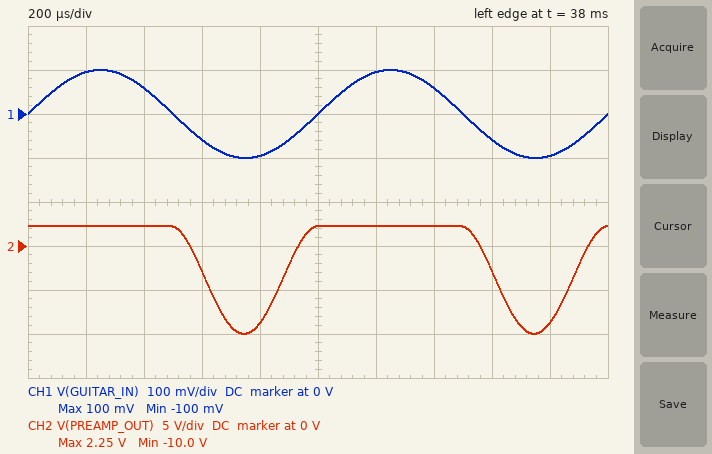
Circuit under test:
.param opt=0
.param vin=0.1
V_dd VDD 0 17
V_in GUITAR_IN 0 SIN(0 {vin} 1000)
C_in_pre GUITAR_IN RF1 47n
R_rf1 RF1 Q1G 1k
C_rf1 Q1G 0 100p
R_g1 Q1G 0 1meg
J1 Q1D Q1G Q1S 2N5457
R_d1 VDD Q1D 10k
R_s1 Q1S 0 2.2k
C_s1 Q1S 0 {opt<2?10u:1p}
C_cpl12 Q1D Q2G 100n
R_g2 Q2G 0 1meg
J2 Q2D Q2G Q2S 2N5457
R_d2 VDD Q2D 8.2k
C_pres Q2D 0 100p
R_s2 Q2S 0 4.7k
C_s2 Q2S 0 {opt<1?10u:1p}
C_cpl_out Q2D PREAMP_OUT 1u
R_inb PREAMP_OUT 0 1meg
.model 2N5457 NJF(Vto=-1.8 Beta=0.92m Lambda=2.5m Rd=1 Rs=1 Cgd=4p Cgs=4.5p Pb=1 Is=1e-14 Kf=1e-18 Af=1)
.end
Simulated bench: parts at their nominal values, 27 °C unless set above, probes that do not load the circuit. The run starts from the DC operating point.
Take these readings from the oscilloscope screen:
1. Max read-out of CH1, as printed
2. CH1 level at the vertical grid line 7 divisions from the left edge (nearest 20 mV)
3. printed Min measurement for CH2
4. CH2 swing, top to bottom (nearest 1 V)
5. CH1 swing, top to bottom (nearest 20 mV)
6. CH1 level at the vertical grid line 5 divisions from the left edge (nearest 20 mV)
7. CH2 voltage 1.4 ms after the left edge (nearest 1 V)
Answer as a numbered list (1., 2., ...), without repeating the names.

1. 100 mV
2. 60 mV
3. -10.0 V
4. 12 V
5. 200 mV
6. 0 V
7. 2 V
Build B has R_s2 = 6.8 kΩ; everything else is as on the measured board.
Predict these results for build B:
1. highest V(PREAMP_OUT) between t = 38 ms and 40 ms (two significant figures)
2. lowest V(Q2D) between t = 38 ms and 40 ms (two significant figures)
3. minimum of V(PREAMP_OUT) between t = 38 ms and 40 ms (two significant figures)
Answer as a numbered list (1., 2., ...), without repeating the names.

1. 1.7 V
2. 7.0 V
3. -8.3 V
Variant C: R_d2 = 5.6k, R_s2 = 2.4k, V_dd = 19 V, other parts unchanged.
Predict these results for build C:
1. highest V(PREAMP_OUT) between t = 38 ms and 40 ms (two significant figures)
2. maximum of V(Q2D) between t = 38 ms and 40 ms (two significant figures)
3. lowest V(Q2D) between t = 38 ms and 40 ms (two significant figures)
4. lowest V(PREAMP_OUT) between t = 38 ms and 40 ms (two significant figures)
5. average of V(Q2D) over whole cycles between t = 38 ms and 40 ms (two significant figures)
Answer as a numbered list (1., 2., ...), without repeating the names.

1. 2.6 V
2. 19 V
3. 6.7 V
4. -9.7 V
5. 15 V
